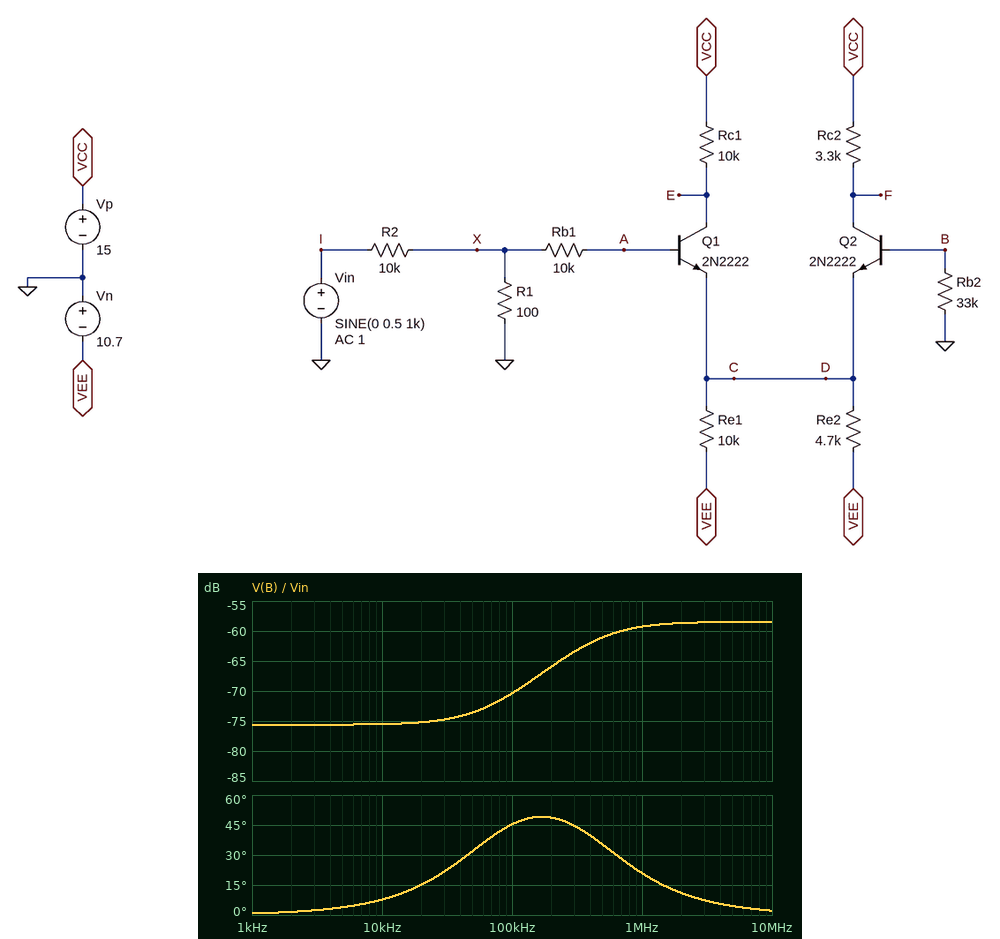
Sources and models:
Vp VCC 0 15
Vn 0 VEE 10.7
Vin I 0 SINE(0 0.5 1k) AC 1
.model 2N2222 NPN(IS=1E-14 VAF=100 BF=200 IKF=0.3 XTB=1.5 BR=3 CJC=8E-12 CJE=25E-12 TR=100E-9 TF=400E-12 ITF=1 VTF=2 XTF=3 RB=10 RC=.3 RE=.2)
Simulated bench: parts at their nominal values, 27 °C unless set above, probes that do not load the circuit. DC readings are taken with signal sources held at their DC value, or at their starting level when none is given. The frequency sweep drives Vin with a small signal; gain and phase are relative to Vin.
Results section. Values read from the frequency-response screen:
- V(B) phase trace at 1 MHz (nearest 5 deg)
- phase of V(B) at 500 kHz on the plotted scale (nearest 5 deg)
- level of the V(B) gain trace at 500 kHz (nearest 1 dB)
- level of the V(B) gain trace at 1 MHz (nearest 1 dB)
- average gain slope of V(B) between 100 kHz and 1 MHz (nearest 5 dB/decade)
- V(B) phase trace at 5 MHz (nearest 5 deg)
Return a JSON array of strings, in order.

["20 deg", "35 deg", "-61 dB", "-59 dB", "10 dB/decade", "5 deg"]
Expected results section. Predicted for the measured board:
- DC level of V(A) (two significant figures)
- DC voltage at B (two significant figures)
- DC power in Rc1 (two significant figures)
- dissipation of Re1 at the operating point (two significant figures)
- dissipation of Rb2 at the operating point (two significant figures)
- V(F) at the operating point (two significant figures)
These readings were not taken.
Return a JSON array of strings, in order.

["-210 mV", "-220 mV", "25 mW", "9.6 mW", "1.5 µW", "10 V"]
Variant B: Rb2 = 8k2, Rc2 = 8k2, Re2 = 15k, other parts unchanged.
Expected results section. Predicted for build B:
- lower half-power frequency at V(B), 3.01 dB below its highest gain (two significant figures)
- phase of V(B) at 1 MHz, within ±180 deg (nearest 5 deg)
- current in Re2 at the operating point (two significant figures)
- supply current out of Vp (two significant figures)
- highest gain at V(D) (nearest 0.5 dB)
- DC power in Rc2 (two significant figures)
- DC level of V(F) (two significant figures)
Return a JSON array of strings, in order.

["13 kHz", "-15 deg", "670 µA", "1.7 mA", "-47.0 dB", "6.4 mW", "7.8 V"]
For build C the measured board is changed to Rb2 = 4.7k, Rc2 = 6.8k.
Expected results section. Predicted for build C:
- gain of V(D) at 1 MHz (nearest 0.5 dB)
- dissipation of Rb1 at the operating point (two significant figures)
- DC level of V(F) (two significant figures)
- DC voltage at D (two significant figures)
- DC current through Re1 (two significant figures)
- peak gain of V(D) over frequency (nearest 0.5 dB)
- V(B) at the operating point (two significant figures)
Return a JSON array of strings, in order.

["-53.0 dB", "330 nW", "1.9 V", "-720 mV", "1.0 mA", "-49.5 dB", "-45 mV"]
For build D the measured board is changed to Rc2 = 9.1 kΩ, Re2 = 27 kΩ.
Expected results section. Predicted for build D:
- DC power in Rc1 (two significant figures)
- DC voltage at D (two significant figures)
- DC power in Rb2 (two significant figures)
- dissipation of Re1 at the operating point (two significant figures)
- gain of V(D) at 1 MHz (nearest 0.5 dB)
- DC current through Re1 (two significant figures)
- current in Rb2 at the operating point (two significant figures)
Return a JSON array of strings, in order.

["8.6 mW", "-700 mV", "130 nW", "10 mW", "-45.0 dB", "1.0 mA", "2.0 µA"]
